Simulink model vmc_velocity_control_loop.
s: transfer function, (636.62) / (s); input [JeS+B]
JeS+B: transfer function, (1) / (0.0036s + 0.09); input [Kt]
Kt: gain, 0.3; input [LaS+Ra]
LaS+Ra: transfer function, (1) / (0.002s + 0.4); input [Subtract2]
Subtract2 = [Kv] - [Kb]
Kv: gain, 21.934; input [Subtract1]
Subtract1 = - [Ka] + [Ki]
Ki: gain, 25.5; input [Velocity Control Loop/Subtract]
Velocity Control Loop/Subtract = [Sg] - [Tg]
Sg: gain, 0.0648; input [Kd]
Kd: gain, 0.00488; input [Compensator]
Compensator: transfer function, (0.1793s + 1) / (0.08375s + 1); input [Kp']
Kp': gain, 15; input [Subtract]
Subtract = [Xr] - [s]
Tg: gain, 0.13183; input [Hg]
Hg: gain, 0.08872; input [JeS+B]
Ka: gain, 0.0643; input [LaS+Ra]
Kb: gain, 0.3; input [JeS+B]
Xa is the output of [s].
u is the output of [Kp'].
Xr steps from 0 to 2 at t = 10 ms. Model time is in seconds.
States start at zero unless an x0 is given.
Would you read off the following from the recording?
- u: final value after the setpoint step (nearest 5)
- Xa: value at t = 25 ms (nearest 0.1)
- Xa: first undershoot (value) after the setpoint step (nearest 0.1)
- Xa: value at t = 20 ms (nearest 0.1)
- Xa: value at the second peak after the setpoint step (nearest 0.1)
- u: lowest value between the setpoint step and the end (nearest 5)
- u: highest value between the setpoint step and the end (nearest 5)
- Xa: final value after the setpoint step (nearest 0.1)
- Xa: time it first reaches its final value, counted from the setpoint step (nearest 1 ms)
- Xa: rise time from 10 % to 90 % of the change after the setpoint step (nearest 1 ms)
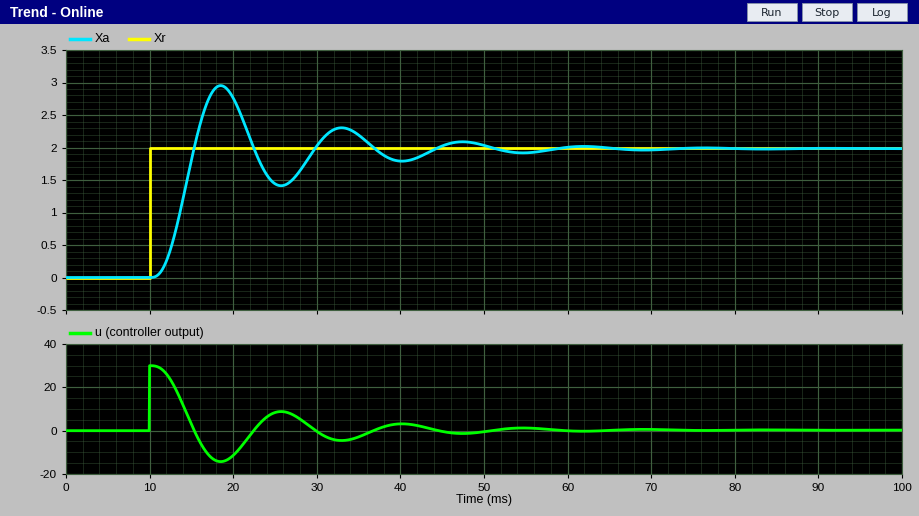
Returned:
0
1.4
1.4
2.8
2.3
-15
30
2.0
5 ms
3 ms
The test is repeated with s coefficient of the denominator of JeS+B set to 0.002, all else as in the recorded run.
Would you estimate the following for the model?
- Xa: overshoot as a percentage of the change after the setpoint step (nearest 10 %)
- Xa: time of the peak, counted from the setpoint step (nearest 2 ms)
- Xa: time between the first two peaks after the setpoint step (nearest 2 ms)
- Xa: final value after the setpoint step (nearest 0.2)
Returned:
40 %
6 ms
10 ms
2.0
